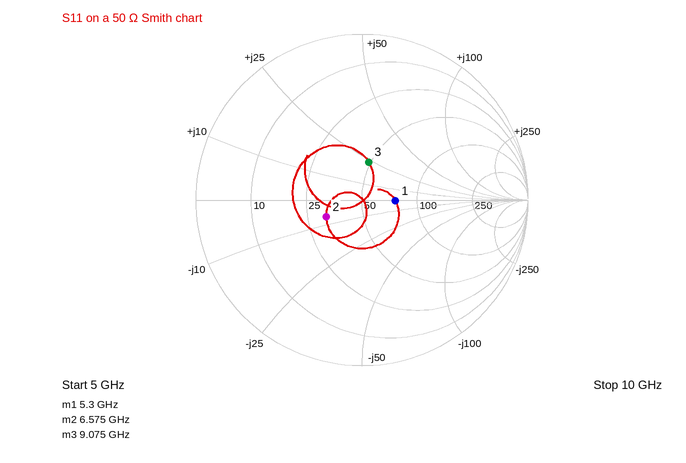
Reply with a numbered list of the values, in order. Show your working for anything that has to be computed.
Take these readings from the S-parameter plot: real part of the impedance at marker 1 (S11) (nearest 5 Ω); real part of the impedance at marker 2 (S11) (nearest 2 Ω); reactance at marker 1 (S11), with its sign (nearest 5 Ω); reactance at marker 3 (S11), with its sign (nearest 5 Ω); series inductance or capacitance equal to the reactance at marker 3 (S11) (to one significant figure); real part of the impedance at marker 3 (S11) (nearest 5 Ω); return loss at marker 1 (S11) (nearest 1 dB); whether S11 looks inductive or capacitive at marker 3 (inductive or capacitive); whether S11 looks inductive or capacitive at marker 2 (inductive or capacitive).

1. 75 Ω
2. 32 Ω
3. 0 Ω
4. +25 Ω
5. L = 25 Ω/(2π × 9.075 GHz) ≈ 438 pH, so 400 pH to one significant figure
6. 50 Ω
7. 14 dB
8. inductive
9. capacitive
